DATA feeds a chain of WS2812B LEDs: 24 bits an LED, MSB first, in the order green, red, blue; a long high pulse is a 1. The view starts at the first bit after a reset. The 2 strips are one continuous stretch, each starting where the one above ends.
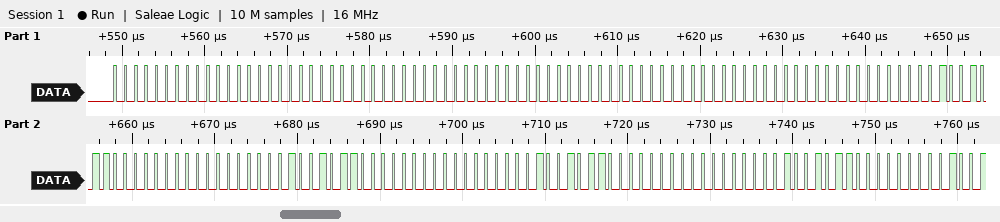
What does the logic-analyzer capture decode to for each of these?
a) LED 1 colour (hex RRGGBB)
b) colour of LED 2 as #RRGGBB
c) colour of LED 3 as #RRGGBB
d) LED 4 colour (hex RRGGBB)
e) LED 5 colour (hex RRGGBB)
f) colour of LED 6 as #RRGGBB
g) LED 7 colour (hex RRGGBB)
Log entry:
#000000
#000000
#000000
#960000
#960000
#960000
#960000
